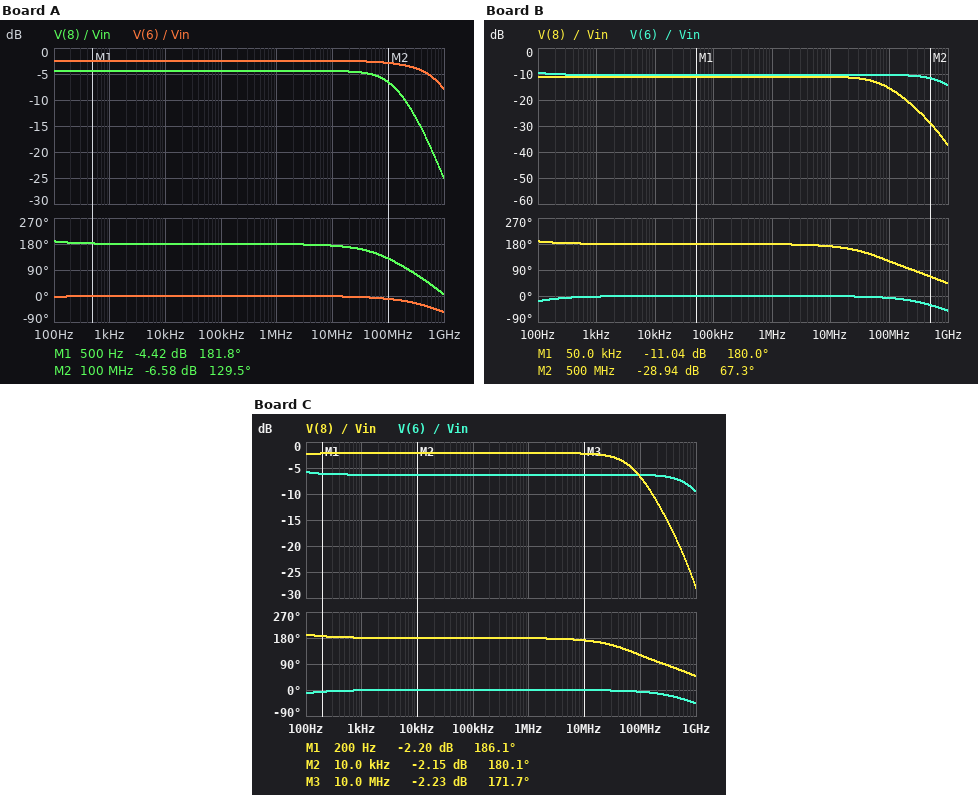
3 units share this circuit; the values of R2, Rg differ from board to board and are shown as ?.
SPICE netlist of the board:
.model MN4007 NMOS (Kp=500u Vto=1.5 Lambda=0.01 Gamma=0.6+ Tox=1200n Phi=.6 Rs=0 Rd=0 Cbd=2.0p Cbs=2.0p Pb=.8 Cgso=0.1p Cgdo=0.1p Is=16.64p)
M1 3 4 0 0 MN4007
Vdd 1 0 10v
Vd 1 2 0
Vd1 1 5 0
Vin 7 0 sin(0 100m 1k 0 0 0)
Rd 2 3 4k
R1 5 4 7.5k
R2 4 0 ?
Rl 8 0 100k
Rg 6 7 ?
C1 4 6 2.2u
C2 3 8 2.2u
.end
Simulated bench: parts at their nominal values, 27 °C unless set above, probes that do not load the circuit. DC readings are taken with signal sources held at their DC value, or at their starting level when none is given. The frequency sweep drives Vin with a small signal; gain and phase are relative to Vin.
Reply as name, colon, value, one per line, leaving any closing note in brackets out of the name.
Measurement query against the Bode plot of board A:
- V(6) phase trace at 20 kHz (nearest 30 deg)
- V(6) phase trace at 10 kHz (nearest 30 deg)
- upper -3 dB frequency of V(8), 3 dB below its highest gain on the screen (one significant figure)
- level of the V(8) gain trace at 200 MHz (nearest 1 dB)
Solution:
V(6) phase trace at 20 kHz: 0 deg
V(6) phase trace at 10 kHz: 0 deg
upper -3 dB frequency of V(8), 3 dB below its highest gain on the screen: 100 MHz
level of the V(8) gain trace at 200 MHz: -10 dB
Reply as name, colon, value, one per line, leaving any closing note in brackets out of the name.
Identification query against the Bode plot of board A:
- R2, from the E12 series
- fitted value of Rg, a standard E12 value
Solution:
R2, from the E12 series: 6.8 kΩ
fitted value of Rg, a standard E12 value: 1.2 kΩ
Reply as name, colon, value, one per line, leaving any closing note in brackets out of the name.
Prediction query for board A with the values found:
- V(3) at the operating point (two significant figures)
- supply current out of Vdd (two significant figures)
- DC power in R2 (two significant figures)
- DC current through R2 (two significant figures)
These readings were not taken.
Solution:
V(3) at the operating point: 1.7 V
supply current out of Vdd: 2.8 mA
DC power in R2: 3.3 mW
DC current through R2: 700 µA
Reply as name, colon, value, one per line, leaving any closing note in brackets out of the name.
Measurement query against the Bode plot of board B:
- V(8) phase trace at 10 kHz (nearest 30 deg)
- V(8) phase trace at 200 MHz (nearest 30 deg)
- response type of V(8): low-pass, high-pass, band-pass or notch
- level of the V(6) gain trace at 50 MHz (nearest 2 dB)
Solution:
V(8) phase trace at 10 kHz: 180 deg
V(8) phase trace at 200 MHz: 90 deg
response type of V(8): low-pass, high-pass, band-pass or notch: low-pass
level of the V(6) gain trace at 50 MHz: -10 dB
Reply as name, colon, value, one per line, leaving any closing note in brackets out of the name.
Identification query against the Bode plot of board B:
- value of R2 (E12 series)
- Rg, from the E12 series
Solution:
value of R2: 1.8 kΩ
Rg, from the E12 series: 3.3 kΩ
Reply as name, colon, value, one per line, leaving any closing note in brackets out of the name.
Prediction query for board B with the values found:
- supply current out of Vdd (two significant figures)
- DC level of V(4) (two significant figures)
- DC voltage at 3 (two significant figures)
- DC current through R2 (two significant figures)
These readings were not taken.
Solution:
supply current out of Vdd: 1.1 mA
DC level of V(4): 1.9 V
DC voltage at 3: 9.8 V
DC current through R2: 1.1 mA
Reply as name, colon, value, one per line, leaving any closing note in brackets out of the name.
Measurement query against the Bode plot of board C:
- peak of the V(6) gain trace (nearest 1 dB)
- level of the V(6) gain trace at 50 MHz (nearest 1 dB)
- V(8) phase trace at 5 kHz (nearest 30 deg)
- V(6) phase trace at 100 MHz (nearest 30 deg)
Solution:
peak of the V(6) gain trace: -6 dB
level of the V(6) gain trace at 50 MHz: -6 dB
V(8) phase trace at 5 kHz: 180 deg
V(6) phase trace at 100 MHz: 0 deg
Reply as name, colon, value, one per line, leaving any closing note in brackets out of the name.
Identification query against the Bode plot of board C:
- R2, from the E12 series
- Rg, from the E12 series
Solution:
R2, from the E12 series: 2.2 kΩ
Rg, from the E12 series: 1.8 kΩ
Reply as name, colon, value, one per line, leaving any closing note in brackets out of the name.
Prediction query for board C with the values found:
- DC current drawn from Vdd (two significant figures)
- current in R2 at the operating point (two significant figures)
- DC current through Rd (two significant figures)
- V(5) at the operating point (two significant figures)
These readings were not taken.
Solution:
DC current drawn from Vdd: 1.2 mA
current in R2 at the operating point: 1.0 mA
DC current through Rd: 160 µA
V(5) at the operating point: 10 V
